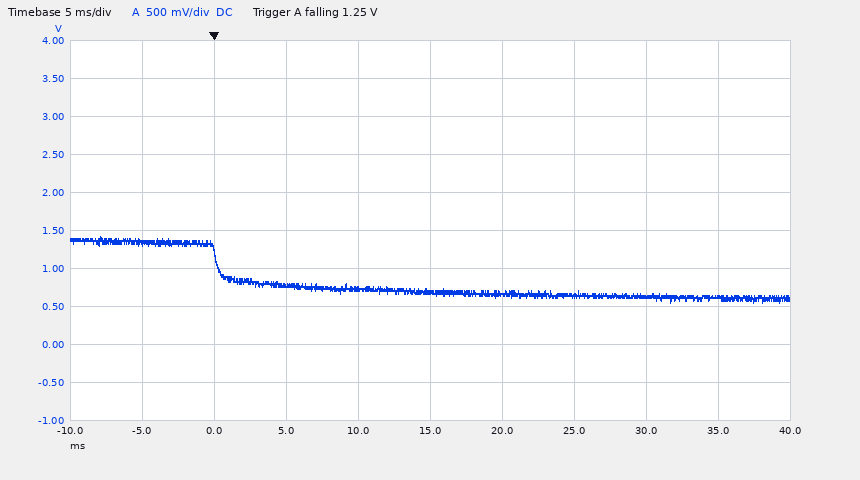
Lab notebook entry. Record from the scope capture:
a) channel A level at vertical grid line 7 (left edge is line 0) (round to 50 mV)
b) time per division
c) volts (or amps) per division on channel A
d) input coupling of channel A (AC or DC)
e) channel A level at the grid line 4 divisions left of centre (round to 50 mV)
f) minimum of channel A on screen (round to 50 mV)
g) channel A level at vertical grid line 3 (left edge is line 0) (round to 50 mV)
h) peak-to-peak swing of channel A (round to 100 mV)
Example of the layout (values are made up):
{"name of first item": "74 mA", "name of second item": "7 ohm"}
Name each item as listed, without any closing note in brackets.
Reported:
{"channel A level at vertical grid line 7 (left edge is line 0)": "650 mV", "time per division": "5 ms", "volts (or amps) per division on channel A": "500 mV", "input coupling of channel A": "DC", "channel A level at the grid line 4 divisions left of centre": "1.35 V", "minimum of channel A on screen": "550 mV", "channel A level at vertical grid line 3 (left edge is line 0)": "800 mV", "peak-to-peak swing of channel A": "900 mV"}
